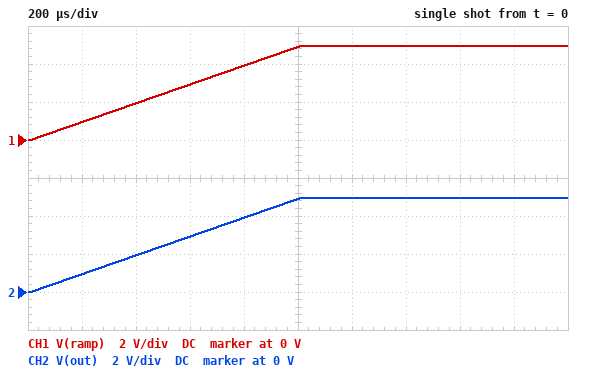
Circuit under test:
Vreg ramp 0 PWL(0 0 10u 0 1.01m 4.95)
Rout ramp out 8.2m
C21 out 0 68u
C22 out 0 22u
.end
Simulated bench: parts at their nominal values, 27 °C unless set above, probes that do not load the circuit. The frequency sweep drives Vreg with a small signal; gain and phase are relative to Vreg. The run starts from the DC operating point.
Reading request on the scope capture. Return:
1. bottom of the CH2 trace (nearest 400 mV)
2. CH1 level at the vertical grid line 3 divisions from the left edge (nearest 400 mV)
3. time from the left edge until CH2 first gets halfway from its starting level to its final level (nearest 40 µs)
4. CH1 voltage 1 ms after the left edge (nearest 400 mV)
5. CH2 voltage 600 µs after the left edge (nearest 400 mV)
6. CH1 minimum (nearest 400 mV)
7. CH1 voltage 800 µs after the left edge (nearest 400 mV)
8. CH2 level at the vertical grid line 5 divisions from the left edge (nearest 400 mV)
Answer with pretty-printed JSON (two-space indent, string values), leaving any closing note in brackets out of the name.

{
  "bottom of the CH2 trace": "0 V",
  "CH1 level at the vertical grid line 3 divisions from the left edge": "2.8 V",
  "time from the left edge until CH2 first gets halfway from its starting level to its final level": "520 µs",
  "CH1 voltage 1 ms after the left edge": "4.8 V",
  "CH2 voltage 600 µs after the left edge": "2.8 V",
  "CH1 minimum": "0 V",
  "CH1 voltage 800 µs after the left edge": "4.0 V",
  "CH2 level at the vertical grid line 5 divisions from the left edge": "4.8 V"
}
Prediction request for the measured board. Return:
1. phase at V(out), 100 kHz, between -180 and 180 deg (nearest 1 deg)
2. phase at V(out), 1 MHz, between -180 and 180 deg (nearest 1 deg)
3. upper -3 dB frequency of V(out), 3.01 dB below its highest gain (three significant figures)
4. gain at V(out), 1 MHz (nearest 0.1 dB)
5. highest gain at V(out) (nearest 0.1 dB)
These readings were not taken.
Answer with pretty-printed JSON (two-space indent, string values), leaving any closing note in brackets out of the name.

{
  "phase at V(out), 100 kHz, between -180 and 180 deg": "-25 deg",
  "phase at V(out), 1 MHz, between -180 and 180 deg": "-78 deg",
  "upper -3 dB frequency of V(out), 3.01 dB below its highest gain": "216 kHz",
  "gain at V(out), 1 MHz": "-13.5 dB",
  "highest gain at V(out)": "0 dB"
}
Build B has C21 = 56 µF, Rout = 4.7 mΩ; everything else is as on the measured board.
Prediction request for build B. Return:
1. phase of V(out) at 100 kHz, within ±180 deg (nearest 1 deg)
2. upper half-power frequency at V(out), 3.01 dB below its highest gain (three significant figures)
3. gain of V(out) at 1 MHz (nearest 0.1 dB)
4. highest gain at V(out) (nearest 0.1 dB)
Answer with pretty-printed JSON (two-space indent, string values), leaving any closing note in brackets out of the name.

{
  "phase of V(out) at 100 kHz, within ±180 deg": "-13 deg",
  "upper half-power frequency at V(out), 3.01 dB below its highest gain": "434 kHz",
  "gain of V(out) at 1 MHz": "-8.0 dB",
  "highest gain at V(out)": "0 dB"
}
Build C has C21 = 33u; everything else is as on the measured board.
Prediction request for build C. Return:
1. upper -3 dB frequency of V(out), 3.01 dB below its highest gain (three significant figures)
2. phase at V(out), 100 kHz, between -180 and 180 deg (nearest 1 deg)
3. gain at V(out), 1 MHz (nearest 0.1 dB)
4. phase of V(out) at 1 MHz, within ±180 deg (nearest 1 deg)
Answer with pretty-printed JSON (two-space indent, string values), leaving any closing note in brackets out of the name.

{
  "upper -3 dB frequency of V(out), 3.01 dB below its highest gain": "353 kHz",
  "phase at V(out), 100 kHz, between -180 and 180 deg": "-16 deg",
  "gain at V(out), 1 MHz": "-9.6 dB",
  "phase of V(out) at 1 MHz, within ±180 deg": "-71 deg"
}
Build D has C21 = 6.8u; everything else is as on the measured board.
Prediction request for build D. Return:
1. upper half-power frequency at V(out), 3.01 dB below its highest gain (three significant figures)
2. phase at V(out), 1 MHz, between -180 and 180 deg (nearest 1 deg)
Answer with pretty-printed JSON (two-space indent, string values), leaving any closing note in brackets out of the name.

{
  "upper half-power frequency at V(out), 3.01 dB below its highest gain": "674 kHz",
  "phase at V(out), 1 MHz, between -180 and 180 deg": "-56 deg"
}
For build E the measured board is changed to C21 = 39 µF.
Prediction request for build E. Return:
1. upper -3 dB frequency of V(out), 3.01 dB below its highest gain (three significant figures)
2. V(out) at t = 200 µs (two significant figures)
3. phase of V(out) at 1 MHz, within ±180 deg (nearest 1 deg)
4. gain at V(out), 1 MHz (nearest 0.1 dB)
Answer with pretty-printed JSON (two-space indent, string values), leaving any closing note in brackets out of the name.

{
  "upper -3 dB frequency of V(out), 3.01 dB below its highest gain": "318 kHz",
  "V(out) at t = 200 µs": "940 mV",
  "phase of V(out) at 1 MHz, within ±180 deg": "-72 deg",
  "gain at V(out), 1 MHz": "-10.4 dB"
}
